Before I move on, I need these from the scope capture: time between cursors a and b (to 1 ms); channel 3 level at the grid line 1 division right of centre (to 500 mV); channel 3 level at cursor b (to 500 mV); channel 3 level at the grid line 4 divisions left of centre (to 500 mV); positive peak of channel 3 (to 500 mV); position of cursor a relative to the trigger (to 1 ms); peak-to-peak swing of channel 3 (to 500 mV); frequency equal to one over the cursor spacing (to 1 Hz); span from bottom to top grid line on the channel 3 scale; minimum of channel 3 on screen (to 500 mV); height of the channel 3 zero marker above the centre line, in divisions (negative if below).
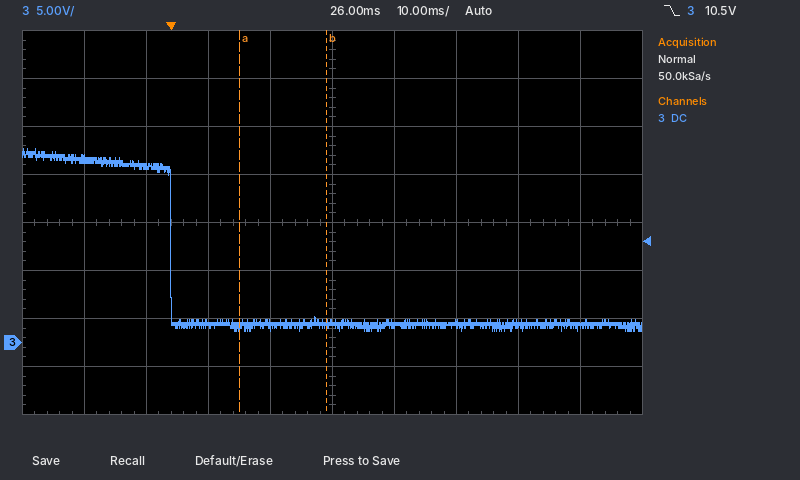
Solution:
14 ms
2.0 V
2.0 V
19.0 V
20.0 V
+11 ms
19.0 V
71 Hz
40 V
1.0 V
-2.5 div
